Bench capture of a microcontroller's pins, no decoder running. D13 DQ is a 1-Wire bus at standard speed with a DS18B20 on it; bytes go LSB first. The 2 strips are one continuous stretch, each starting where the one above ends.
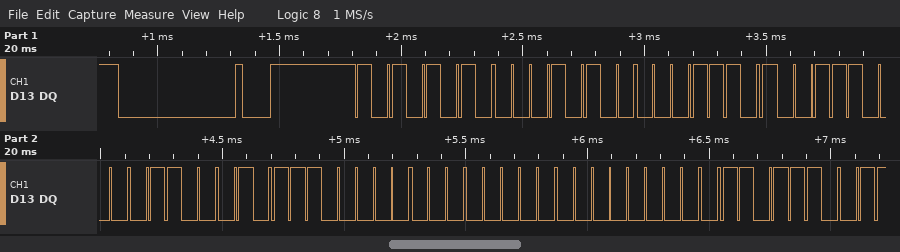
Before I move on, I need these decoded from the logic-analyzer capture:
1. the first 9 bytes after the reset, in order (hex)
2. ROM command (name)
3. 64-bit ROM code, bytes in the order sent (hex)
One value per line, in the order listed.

55 28 B8 1C 46 07 00 00 76
Match ROM
28 B8 1C 46 07 00 00 76
